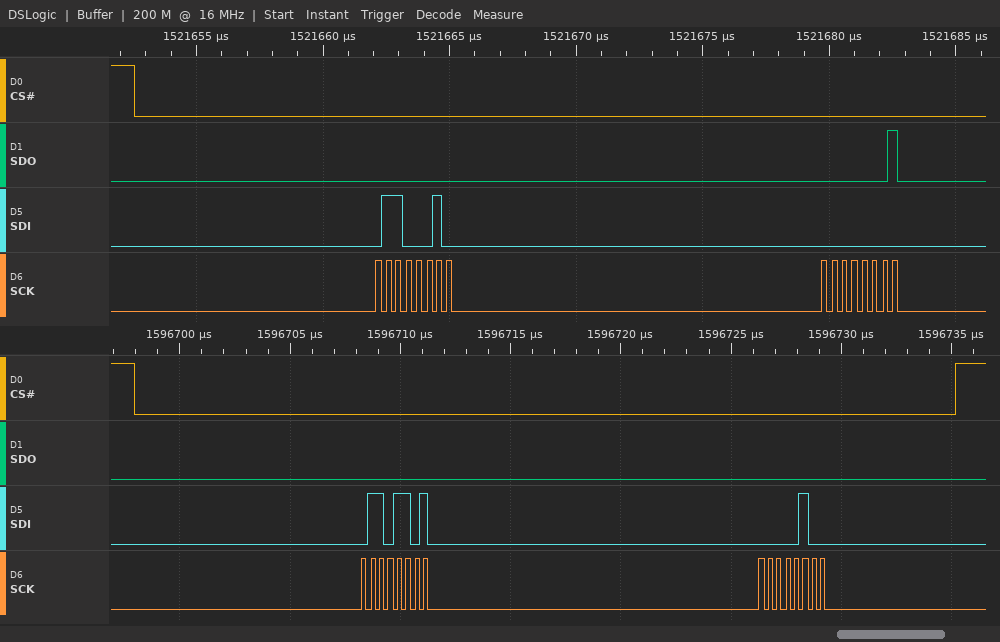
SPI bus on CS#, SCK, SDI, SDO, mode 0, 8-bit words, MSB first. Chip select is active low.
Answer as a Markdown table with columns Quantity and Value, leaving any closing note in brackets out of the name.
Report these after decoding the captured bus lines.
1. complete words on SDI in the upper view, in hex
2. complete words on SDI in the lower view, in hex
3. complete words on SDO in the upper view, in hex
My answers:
| Quantity | Value |
|---|---|
| complete words on SDI in the upper view, in hex | 62, 00 |
| complete words on SDI in the lower view, in hex | 6D, 04 |
| complete words on SDO in the upper view, in hex | 00, 01 |
